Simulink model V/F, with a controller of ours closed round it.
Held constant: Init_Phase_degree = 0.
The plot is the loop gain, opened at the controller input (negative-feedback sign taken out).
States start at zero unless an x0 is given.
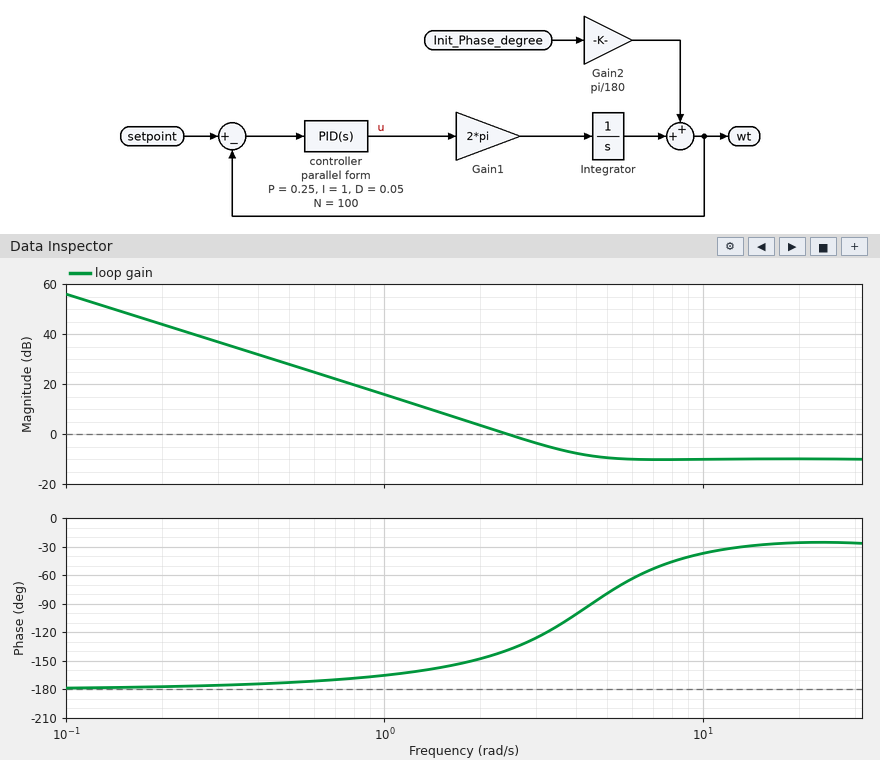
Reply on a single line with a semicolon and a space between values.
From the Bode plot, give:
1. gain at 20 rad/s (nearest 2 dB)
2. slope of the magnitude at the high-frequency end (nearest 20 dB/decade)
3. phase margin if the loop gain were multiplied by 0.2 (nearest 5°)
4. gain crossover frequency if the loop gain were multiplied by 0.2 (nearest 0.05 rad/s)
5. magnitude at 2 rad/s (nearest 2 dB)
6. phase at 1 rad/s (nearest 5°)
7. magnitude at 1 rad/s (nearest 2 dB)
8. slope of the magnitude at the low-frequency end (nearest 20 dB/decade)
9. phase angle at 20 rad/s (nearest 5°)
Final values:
-10 dB; 0 dB/decade; 15°; 1.10 rad/s; 4 dB; -165°; 16 dB; -40 dB/decade; -25°
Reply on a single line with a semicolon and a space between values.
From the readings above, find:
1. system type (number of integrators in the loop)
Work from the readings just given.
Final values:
2
